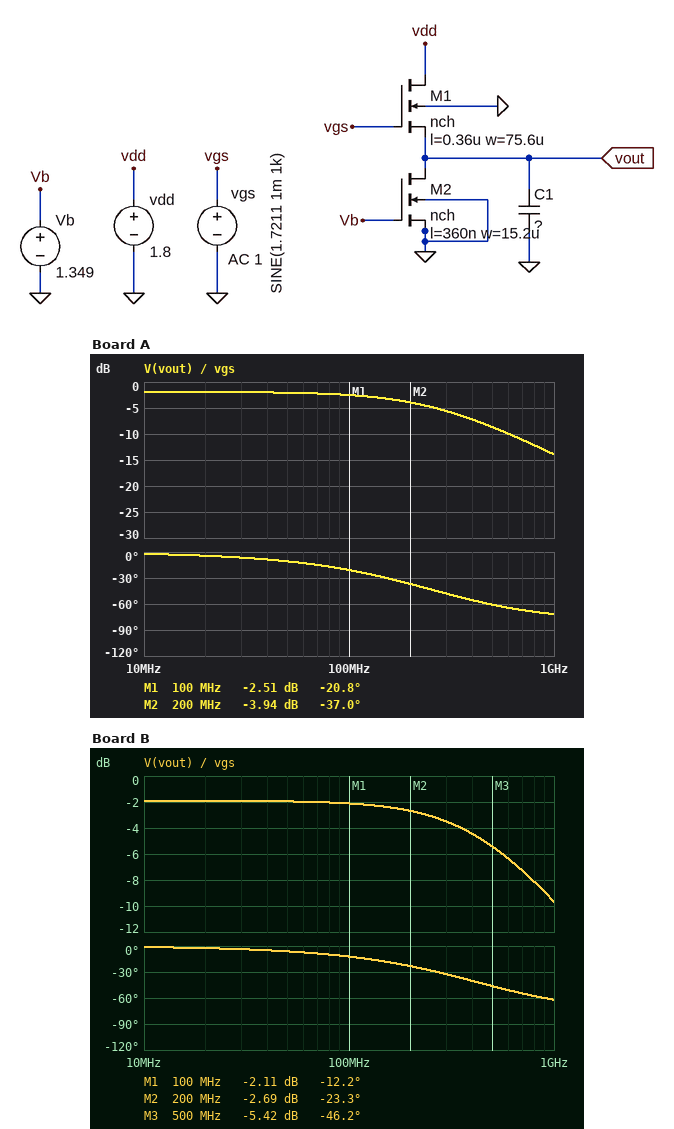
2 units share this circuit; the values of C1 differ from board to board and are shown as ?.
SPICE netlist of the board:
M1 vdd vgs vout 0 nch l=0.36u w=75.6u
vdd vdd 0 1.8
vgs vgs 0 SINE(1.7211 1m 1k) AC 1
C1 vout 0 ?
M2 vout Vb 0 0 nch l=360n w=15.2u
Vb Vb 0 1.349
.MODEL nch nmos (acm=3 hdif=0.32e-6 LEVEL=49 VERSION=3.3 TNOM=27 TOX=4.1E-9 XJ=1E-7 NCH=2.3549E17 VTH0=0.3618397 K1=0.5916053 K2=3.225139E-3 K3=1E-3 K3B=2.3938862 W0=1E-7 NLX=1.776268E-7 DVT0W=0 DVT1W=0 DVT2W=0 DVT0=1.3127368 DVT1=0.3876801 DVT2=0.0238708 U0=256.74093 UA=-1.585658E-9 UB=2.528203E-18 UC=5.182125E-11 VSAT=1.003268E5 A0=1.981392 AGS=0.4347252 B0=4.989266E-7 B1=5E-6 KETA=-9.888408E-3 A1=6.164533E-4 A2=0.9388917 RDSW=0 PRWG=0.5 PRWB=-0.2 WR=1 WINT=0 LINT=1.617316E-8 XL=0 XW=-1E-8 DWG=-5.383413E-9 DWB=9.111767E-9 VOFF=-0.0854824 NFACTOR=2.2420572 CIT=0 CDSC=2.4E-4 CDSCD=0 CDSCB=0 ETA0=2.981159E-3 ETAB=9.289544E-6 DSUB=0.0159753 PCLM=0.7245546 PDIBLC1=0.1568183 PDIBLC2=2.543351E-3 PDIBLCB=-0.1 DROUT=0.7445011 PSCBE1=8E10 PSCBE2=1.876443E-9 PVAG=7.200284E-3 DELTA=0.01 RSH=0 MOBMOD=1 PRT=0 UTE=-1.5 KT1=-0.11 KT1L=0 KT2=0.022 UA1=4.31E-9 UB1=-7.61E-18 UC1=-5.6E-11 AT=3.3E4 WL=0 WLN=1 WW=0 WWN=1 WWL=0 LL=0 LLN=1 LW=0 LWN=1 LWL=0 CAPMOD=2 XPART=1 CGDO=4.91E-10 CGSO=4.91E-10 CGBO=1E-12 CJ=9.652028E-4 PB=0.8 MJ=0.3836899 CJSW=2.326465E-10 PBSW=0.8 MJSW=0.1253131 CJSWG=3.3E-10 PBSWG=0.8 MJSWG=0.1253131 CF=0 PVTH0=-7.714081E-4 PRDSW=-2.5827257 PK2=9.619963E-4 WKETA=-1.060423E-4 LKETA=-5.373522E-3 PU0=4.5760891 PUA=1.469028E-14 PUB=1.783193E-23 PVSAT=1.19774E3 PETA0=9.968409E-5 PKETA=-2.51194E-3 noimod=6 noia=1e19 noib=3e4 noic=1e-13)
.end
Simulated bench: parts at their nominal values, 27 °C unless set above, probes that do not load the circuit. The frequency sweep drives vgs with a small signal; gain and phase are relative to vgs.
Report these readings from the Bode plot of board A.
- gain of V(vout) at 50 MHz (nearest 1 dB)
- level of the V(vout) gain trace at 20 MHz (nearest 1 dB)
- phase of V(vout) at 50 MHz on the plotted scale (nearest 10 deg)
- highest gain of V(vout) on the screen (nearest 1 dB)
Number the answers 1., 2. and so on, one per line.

1. -2 dB
2. -2 dB
3. -10 deg
4. -2 dB
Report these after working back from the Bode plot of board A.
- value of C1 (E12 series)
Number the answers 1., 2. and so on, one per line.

1. 12 pF
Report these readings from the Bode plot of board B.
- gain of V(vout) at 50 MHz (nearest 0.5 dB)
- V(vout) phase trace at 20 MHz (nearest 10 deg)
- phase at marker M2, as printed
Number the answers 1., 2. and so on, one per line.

1. -2.0 dB
2. 0 deg
3. -23.3 deg
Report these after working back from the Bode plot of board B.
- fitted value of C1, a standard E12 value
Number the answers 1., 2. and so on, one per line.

1. 6.8 pF
